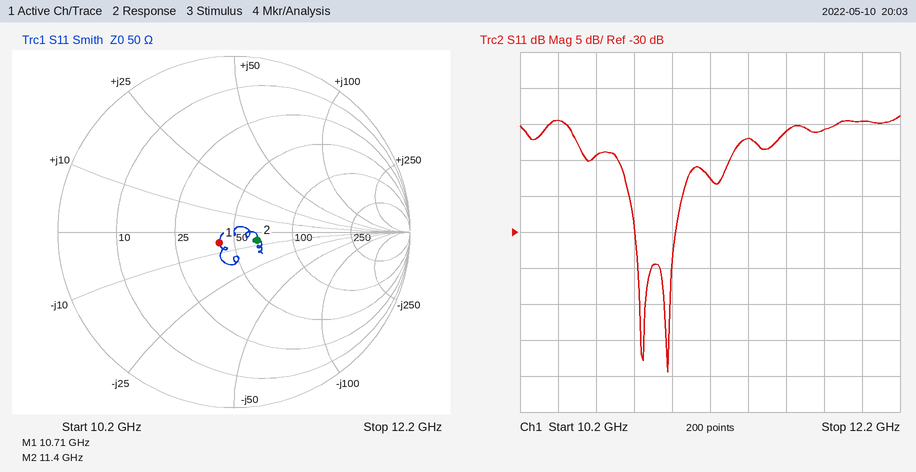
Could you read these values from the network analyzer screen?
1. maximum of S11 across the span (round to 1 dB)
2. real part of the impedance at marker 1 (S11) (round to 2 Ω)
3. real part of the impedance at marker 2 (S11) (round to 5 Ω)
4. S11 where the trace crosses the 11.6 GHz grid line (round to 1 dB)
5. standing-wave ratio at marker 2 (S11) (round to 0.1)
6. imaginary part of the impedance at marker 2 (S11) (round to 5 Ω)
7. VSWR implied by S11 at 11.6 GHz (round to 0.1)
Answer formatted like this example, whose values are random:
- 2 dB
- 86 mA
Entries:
- -14 dB
- 42 Ω
- 65 Ω
- -16 dB
- 1.3
- -5 Ω
- 1.4
